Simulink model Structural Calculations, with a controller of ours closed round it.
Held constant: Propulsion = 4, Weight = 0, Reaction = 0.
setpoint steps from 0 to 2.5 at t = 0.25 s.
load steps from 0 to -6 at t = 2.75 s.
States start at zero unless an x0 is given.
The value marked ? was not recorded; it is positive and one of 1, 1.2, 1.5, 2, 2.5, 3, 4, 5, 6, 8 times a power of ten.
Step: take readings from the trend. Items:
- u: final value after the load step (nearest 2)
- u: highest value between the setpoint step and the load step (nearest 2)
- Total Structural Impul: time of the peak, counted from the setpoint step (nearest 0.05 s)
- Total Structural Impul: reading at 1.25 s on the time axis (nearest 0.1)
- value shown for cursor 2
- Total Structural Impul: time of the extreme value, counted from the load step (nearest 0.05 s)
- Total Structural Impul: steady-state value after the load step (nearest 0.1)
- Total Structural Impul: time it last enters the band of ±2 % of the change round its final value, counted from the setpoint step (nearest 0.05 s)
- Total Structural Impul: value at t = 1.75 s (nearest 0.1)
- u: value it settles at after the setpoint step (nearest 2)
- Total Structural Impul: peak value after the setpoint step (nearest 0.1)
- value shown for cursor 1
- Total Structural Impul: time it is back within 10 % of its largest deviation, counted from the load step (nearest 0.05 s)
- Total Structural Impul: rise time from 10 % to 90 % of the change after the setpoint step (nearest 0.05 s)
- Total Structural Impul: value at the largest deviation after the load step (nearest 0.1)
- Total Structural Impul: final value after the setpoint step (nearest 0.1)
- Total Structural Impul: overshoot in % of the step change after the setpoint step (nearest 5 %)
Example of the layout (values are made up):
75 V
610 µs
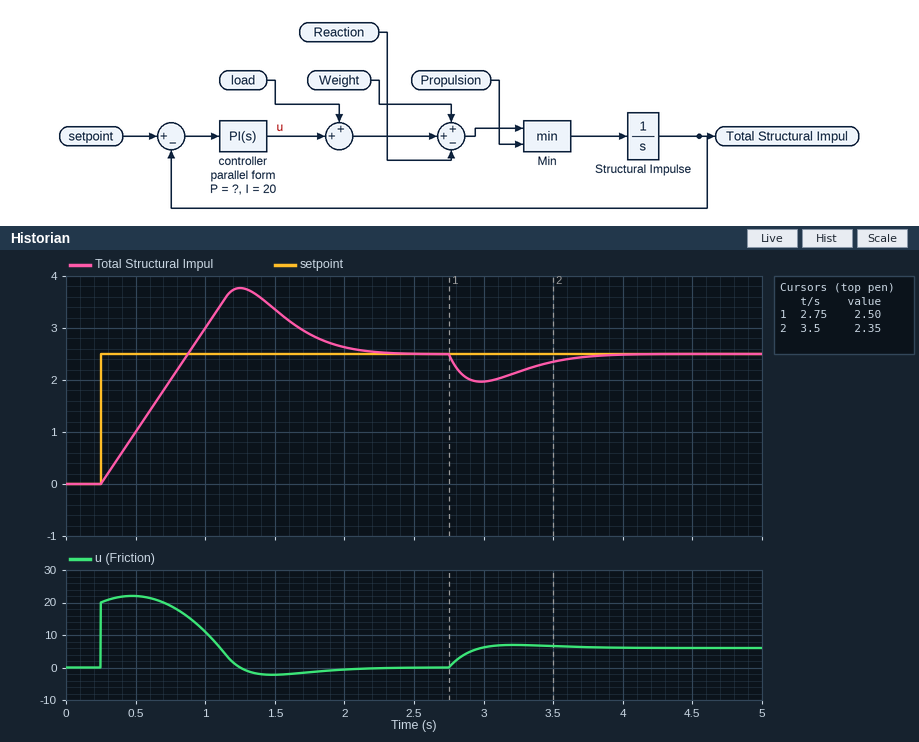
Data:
6
22
1.00 s
3.8
2.35
0.25 s
2.5
1.95 s
2.9
0
3.8
2.50
1.00 s
0.50 s
2.0
2.5
50 %
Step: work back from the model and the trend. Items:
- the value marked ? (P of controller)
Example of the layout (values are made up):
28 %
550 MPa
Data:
8
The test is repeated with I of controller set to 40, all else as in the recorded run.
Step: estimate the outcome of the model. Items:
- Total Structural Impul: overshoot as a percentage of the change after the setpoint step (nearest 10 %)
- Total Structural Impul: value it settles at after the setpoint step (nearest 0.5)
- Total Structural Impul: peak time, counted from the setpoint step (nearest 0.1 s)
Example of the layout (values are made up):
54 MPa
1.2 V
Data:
70 %
2.5
1.1 s
